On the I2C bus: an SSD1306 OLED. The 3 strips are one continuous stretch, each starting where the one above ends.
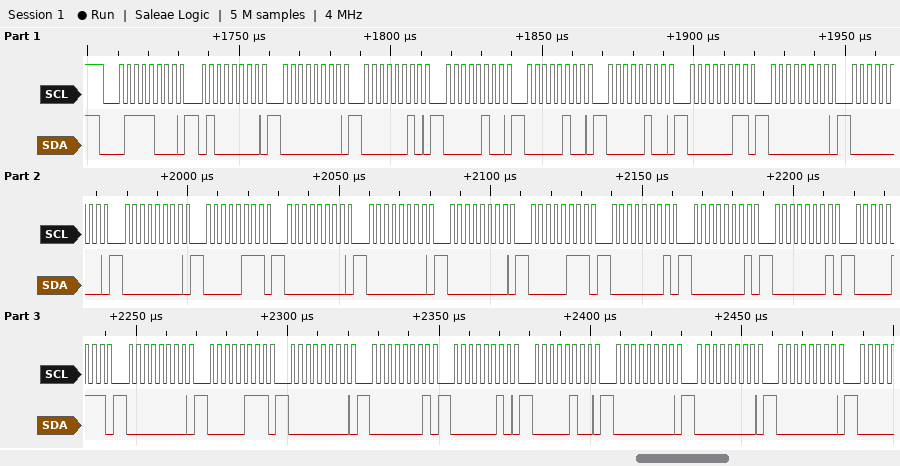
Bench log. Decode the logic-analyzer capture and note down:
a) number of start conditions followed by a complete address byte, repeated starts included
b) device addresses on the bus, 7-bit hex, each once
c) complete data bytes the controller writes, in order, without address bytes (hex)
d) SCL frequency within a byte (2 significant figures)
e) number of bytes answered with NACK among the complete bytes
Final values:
1
0x3C
40 00 02 04 04 04 03 00 00 00 07 00 00 00 07 01 01 01 07 00 07 00 01 02 04 00 00 00
400 kHz
0
